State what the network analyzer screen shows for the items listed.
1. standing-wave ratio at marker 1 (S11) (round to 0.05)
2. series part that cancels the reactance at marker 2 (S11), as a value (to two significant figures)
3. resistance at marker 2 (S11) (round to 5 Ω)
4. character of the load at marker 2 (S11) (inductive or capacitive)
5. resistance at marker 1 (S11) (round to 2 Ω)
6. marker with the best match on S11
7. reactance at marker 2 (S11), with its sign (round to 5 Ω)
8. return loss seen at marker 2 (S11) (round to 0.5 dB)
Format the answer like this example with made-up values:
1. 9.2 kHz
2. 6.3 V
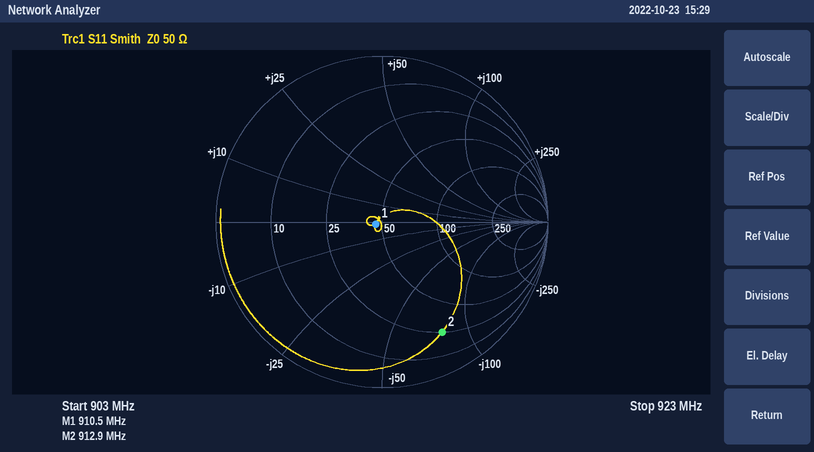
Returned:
1. 1.10
2. 14 nH
3. 25 Ω
4. capacitive
5. 46 Ω
6. marker 1
7. -80 Ω
8. 2.5 dB
